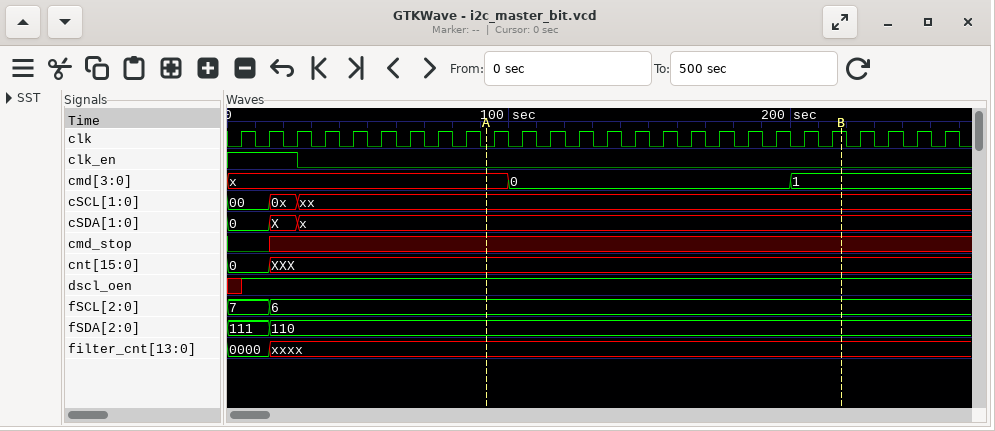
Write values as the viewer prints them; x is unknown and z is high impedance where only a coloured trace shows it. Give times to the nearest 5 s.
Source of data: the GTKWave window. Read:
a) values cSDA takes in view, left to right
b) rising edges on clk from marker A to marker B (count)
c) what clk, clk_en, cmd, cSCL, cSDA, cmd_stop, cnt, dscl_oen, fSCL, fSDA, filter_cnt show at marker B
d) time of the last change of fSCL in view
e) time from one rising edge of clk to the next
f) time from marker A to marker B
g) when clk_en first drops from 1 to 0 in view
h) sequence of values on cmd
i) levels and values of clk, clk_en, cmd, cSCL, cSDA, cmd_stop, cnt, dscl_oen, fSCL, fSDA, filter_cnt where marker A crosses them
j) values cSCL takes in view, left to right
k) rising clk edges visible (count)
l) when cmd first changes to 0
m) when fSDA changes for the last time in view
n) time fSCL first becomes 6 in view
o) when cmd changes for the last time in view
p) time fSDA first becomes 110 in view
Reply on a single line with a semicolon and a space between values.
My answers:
0, X, x; 13; clk=1, clk_en=0, cmd=1, cSCL=xx, cSDA=x, cmd_stop=x, cnt=XXX, dscl_oen=1, fSCL=6, fSDA=110, filter_cnt=xxxx; 15 s; 10 s; 125 s; 25 s; x, 0, 1; clk=0, clk_en=0, cmd=x, cSCL=xx, cSDA=x, cmd_stop=x, cnt=XXX, dscl_oen=1, fSCL=6, fSDA=110, filter_cnt=xxxx; 00, 0x, xx; 26; 100 s; 15 s; 15 s; 200 s; 15 s
